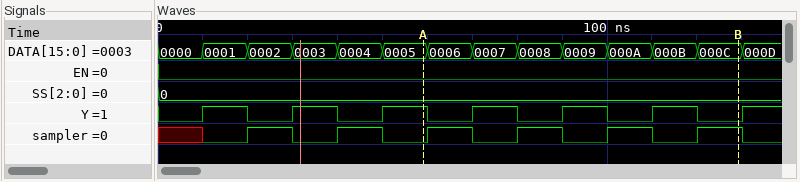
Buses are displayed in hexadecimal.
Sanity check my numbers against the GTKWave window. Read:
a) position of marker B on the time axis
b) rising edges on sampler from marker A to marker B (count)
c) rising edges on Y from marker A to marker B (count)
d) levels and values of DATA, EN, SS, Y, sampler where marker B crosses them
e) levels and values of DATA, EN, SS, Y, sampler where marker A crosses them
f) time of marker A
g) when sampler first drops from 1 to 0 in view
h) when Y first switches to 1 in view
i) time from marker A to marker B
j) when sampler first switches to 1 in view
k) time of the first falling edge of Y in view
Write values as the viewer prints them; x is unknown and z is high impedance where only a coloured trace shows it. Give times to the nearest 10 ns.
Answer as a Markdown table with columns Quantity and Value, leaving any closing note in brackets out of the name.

| Quantity | Value |
|---|---|
| position of marker B on the time axis | 130 ns |
| rising edges on sampler from marker A to marker B | 4 |
| rising edges on Y from marker A to marker B | 3 |
| levels and values of DATA, EN, SS, Y, sampler where marker B crosses them | DATA=000C, EN=0, SS=0, Y=0, sampler=1 |
| levels and values of DATA, EN, SS, Y, sampler where marker A crosses them | DATA=0005, EN=0, SS=0, Y=1, sampler=0 |
| time of marker A | 60 ns |
| when sampler first drops from 1 to 0 in view | 30 ns |
| when Y first switches to 1 in view | 10 ns |
| time from marker A to marker B | 70 ns |
| when sampler first switches to 1 in view | 20 ns |
| time of the first falling edge of Y in view | 20 ns |
